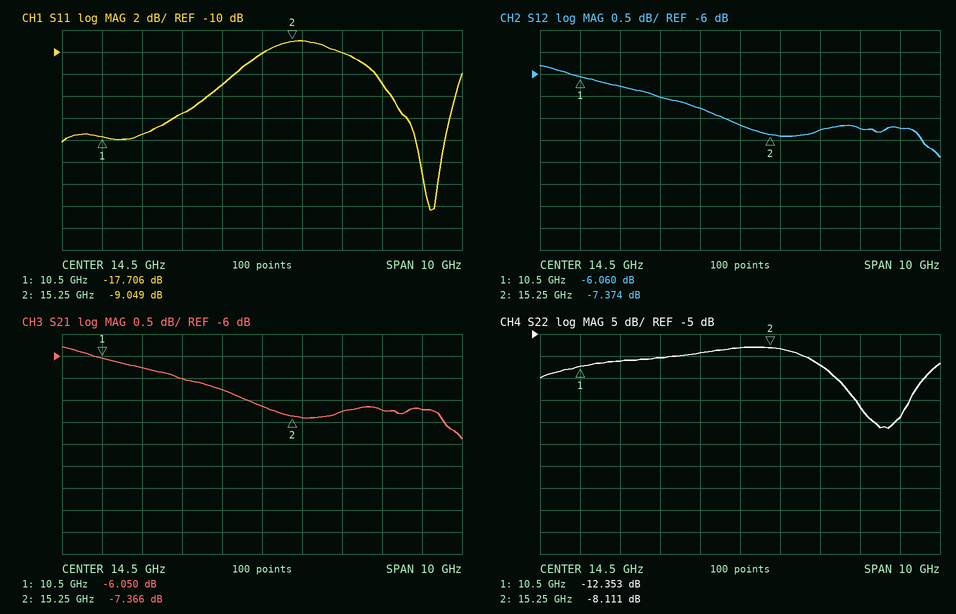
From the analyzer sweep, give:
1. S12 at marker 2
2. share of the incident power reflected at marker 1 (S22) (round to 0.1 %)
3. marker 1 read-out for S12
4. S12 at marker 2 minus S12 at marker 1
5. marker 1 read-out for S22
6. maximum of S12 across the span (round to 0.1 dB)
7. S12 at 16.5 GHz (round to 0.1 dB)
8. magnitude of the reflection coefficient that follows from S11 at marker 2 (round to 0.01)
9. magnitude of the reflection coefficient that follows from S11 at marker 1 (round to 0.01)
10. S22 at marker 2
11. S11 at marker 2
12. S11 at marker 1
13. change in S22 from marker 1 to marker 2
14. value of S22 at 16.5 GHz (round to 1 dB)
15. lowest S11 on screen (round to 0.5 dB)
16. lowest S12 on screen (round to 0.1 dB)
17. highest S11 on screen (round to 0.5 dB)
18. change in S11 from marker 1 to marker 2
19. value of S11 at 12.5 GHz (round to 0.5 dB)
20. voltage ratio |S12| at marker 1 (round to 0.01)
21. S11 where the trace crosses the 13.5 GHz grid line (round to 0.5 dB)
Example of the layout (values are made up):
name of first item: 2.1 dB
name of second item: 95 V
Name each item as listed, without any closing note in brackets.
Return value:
S12 at marker 2: -7.374 dB
share of the incident power reflected at marker 1 (S22): 5.8 %
marker 1 read-out for S12: -6.060 dB
S12 at marker 2 minus S12 at marker 1: -1.314 dB
marker 1 read-out for S22: -12.353 dB
maximum of S12 across the span: -5.8 dB
S12 at 16.5 GHz: -7.3 dB
magnitude of the reflection coefficient that follows from S11 at marker 2: 0.35
magnitude of the reflection coefficient that follows from S11 at marker 1: 0.13
S22 at marker 2: -8.111 dB
S11 at marker 2: -9.049 dB
S11 at marker 1: -17.706 dB
change in S22 from marker 1 to marker 2: 4.242 dB
value of S22 at 16.5 GHz: -12 dB
lowest S11 on screen: -24.5 dB
lowest S12 on screen: -7.9 dB
highest S11 on screen: -9.0 dB
change in S11 from marker 1 to marker 2: 8.657 dB
value of S11 at 12.5 GHz: -15.5 dB
voltage ratio |S12| at marker 1: 0.50
S11 where the trace crosses the 13.5 GHz grid line: -13.0 dB
